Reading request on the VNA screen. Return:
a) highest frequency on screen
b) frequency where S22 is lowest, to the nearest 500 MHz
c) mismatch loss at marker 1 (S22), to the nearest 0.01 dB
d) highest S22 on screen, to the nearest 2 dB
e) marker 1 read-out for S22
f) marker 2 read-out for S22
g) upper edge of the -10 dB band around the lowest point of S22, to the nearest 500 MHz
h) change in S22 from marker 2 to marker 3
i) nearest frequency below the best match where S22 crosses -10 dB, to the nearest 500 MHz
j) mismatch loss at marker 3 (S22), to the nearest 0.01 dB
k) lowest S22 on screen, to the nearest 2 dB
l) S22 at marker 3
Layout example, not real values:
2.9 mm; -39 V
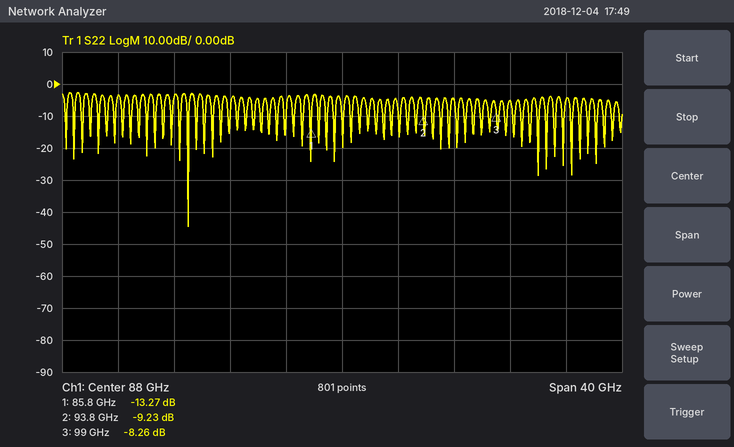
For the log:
108 GHz; 77.0 GHz; 0.21 dB; -2 dB; -13.27 dB; -9.23 dB; 77.0 GHz; 0.97 dB; 77.0 GHz; 0.70 dB; -44 dB; -8.26 dB
